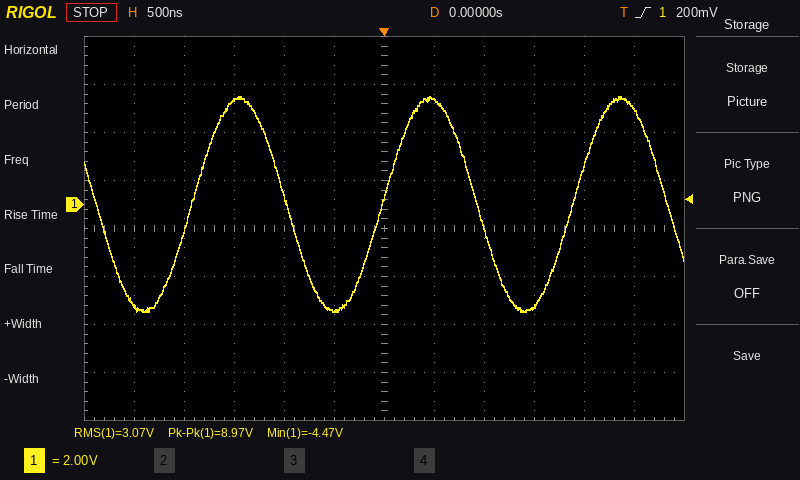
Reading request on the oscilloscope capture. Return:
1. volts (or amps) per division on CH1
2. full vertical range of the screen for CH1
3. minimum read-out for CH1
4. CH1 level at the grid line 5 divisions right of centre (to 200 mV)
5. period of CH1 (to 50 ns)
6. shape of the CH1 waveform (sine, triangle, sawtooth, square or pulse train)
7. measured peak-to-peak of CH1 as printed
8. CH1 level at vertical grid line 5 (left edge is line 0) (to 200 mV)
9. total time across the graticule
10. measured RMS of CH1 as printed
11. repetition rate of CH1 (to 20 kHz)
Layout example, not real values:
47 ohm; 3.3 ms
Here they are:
2 V; 16 V; -4.47 V; 4.0 V; 1.90 µs; sine; 8.97 V; -4.4 V; 6 µs; 3.07 V; 520 kHz
